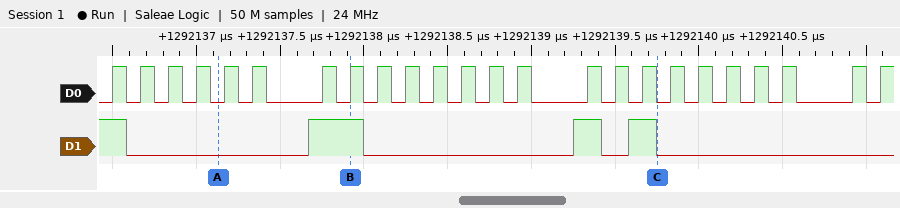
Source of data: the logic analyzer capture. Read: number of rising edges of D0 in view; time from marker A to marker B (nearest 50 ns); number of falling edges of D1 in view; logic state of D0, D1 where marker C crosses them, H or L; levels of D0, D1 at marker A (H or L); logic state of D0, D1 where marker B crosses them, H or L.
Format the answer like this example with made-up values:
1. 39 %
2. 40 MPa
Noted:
1. 24
2. 800 ns
3. 4
4. D0=L, D1=L
5. D0=L, D1=L
6. D0=H, D1=H
